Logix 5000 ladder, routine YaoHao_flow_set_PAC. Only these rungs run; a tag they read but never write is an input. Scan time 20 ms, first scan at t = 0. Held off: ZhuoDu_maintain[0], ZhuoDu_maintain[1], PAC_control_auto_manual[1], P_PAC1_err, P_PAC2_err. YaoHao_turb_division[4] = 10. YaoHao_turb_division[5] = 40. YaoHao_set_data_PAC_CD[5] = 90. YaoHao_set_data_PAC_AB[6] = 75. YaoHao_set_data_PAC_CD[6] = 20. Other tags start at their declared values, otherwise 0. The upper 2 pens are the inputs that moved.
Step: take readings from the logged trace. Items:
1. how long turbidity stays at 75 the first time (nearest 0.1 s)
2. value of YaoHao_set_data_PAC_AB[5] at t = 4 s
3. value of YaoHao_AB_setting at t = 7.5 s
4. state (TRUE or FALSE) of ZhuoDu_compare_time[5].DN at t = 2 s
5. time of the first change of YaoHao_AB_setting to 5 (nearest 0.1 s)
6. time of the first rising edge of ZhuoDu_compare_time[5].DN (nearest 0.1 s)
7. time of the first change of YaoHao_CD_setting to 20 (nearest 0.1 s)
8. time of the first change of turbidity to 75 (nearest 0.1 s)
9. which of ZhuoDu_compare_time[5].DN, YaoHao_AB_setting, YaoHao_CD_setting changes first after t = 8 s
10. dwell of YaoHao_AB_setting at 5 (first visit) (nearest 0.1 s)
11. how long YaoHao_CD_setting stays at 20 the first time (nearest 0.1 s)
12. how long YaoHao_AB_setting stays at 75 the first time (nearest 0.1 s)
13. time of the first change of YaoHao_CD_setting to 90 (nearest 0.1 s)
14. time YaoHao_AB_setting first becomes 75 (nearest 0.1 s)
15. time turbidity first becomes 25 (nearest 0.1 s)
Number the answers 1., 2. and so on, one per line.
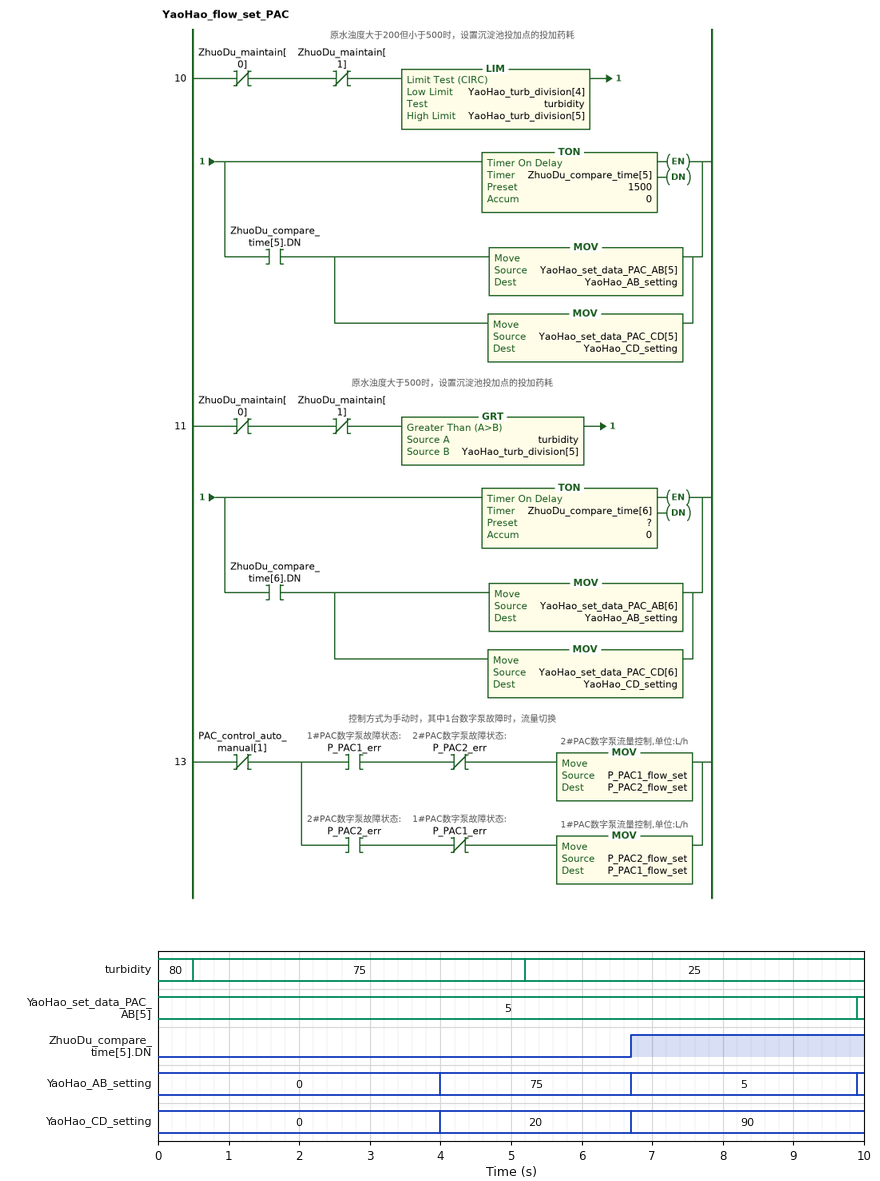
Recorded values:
1. 4.7 s
2. 5
3. 5
4. FALSE
5. 6.7 s
6. 6.7 s
7. 4.0 s
8. 0.5 s
9. YaoHao_AB_setting
10. 3.2 s
11. 2.7 s
12. 2.7 s
13. 6.7 s
14. 4.0 s
15. 5.2 s
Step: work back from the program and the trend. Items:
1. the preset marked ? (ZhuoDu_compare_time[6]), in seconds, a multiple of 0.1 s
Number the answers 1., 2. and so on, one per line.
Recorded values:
1. 4.0 s
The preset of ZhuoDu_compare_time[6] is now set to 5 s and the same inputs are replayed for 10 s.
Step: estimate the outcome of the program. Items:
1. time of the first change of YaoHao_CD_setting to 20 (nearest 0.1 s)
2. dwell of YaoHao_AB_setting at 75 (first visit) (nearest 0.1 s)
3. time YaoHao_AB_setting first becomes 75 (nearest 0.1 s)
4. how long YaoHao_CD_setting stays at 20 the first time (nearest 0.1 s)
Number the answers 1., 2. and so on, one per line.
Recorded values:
1. 5.0 s
2. 1.7 s
3. 5.0 s
4. 1.7 s
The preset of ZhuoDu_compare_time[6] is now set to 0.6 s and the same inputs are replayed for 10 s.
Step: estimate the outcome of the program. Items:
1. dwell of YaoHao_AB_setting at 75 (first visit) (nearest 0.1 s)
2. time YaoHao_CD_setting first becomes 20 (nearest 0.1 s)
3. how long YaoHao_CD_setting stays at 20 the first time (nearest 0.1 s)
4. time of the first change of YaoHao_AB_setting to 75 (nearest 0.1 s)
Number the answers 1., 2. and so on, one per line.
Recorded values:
1. 6.1 s
2. 0.6 s
3. 6.1 s
4. 0.6 s
